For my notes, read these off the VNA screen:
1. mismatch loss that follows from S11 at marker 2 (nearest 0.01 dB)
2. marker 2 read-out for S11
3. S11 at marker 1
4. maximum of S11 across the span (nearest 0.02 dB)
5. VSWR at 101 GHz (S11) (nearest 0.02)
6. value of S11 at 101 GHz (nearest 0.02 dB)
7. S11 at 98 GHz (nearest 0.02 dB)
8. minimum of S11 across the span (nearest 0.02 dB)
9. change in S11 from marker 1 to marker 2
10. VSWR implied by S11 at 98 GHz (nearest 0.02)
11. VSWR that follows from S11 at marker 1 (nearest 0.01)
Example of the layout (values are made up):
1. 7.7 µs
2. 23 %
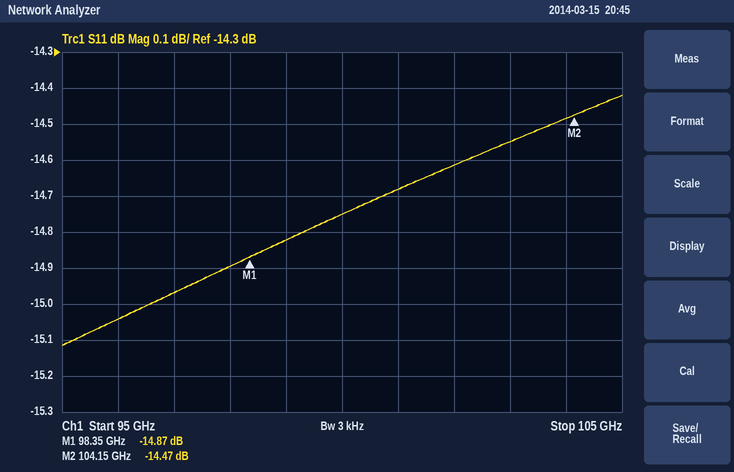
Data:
1. 0.16 dB
2. -14.47 dB
3. -14.87 dB
4. -14.42 dB
5. 1.46
6. -14.68 dB
7. -14.90 dB
8. -15.12 dB
9. 0.40 dB
10. 1.44
11. 1.44
